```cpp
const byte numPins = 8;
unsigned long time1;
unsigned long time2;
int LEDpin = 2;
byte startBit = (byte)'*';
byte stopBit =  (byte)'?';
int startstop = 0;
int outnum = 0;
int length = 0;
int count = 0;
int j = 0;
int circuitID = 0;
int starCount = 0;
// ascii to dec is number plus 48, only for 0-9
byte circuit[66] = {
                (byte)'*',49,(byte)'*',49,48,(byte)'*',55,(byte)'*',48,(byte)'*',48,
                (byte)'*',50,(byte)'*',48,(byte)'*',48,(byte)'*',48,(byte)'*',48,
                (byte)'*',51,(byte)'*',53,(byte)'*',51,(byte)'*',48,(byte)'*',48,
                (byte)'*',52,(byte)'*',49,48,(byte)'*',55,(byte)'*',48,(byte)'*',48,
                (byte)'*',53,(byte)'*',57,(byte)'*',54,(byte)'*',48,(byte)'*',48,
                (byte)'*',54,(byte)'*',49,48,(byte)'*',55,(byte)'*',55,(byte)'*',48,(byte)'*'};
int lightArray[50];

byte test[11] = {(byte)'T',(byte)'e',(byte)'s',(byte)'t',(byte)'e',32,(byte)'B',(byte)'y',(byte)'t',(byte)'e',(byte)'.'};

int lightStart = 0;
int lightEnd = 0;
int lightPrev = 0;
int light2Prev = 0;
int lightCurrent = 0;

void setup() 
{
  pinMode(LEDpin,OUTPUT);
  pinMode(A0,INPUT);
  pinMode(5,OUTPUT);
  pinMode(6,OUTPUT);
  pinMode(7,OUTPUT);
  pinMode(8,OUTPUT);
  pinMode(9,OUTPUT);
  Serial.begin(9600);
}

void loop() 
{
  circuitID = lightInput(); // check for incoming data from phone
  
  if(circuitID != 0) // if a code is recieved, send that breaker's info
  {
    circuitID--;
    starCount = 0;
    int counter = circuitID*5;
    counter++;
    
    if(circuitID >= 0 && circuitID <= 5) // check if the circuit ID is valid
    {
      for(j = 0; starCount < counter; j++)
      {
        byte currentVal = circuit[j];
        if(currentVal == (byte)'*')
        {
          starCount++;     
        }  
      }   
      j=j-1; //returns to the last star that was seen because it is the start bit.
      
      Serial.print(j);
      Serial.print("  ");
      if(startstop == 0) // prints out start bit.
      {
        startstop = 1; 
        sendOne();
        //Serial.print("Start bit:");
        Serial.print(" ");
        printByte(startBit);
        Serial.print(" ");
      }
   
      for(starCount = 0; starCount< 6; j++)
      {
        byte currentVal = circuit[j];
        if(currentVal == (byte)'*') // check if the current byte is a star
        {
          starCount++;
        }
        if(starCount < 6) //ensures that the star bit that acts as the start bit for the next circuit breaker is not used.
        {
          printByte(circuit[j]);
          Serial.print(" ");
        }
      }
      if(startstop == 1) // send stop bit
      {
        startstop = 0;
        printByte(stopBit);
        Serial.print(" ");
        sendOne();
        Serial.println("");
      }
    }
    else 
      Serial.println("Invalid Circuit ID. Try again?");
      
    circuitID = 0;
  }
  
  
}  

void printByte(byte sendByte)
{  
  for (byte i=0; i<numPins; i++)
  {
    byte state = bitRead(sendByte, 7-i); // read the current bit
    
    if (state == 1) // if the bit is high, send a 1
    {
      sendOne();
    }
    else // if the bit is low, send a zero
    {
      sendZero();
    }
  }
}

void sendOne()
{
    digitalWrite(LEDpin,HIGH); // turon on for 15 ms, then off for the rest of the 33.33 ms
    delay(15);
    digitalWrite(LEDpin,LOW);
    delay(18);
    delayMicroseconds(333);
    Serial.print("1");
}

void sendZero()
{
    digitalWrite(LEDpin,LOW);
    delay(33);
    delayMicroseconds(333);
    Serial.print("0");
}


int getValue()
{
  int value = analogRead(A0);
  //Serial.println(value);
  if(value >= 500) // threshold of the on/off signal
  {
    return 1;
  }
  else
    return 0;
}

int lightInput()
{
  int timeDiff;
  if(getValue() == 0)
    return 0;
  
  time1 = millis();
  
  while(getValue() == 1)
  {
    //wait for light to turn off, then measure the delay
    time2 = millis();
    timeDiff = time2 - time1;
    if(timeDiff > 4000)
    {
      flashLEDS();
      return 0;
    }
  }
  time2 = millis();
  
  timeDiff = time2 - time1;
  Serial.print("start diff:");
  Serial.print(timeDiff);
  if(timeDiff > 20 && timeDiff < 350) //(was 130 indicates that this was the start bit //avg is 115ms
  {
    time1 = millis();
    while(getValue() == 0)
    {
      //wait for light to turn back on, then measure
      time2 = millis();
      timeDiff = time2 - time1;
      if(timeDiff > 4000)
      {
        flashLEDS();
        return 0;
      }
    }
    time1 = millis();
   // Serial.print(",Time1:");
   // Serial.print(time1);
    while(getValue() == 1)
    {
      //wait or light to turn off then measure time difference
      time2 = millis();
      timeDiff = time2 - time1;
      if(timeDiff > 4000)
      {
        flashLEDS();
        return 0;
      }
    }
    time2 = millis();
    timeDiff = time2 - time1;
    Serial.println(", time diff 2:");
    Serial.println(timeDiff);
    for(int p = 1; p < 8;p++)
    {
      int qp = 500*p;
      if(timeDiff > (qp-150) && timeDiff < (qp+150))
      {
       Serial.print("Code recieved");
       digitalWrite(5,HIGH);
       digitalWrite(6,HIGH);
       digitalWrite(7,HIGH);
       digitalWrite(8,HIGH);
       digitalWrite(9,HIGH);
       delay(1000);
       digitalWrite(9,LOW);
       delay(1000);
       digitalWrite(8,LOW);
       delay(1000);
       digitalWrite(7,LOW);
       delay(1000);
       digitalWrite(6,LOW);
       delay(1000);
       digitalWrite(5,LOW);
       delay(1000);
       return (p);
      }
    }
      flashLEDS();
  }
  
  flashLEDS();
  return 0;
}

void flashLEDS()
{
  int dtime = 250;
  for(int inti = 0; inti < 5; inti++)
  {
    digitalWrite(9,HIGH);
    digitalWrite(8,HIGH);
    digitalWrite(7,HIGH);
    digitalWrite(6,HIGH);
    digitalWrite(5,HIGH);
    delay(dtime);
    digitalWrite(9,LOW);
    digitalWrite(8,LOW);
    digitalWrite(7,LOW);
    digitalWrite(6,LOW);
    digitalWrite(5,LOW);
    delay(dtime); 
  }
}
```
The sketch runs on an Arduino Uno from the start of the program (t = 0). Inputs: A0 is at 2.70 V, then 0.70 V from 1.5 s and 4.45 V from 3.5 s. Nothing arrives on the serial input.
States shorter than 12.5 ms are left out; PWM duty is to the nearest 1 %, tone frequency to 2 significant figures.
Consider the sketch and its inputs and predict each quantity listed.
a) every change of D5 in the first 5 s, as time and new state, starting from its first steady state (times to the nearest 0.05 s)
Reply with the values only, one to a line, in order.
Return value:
0 s low; 1.5 s high; 1.75 s low; 2 s high; 2.25 s low; 2.5 s high; 2.75 s low; 3 s high; 3.25 s low; 3.5 s high; 3.75 s low
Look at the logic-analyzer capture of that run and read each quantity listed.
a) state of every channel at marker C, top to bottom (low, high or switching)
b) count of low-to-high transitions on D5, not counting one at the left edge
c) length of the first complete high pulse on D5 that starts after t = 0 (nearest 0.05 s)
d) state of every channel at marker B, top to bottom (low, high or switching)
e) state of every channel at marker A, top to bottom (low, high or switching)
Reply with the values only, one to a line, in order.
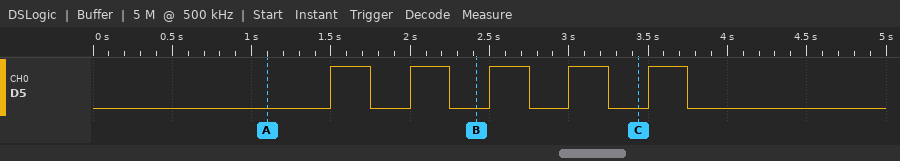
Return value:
D5 low
5
0.25 s
D5 low
D5 low
